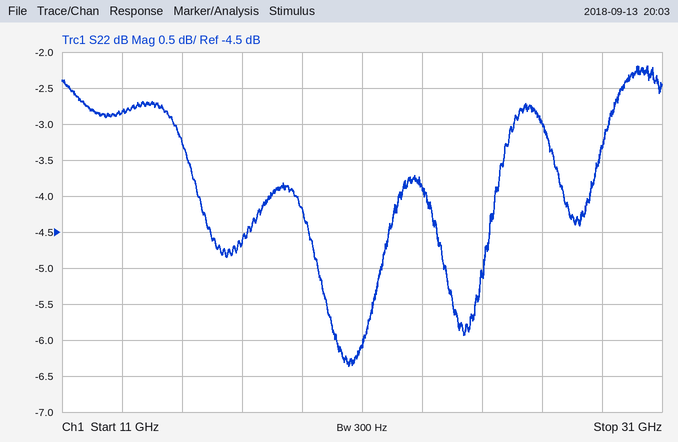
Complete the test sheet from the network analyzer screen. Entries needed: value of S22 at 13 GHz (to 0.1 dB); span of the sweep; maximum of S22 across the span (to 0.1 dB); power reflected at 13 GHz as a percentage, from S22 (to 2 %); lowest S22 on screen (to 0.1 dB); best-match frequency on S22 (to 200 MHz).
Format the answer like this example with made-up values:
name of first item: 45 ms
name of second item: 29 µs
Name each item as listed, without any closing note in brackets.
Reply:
value of S22 at 13 GHz: -2.8 dB
span of the sweep: 20 GHz
maximum of S22 across the span: -2.2 dB
power reflected at 13 GHz as a percentage, from S22: 52 %
lowest S22 on screen: -6.4 dB
best-match frequency on S22: 20.6 GHz
